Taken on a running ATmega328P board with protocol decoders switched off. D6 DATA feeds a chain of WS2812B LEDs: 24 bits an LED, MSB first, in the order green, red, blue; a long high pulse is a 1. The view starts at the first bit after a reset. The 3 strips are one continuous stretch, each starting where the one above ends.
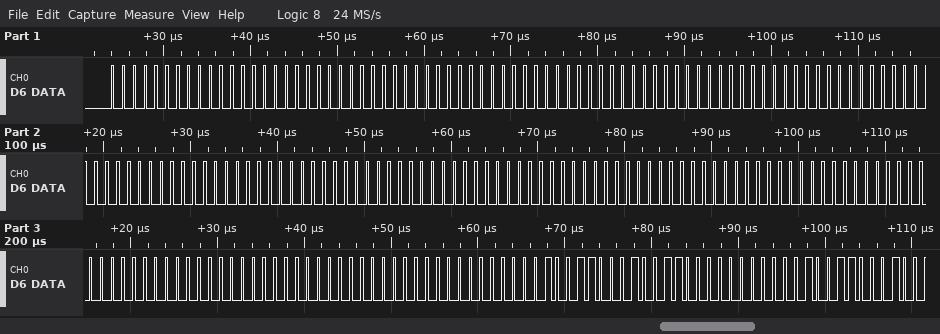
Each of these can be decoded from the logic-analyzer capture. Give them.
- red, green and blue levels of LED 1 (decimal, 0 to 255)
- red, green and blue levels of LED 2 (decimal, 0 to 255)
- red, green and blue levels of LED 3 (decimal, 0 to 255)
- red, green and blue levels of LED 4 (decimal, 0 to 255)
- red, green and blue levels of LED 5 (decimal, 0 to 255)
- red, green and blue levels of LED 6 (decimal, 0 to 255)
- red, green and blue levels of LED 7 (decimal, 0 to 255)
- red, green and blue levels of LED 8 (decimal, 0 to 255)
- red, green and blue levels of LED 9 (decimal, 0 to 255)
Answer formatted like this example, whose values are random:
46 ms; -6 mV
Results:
0, 0, 0; 0, 0, 0; 0, 0, 0; 0, 0, 0; 0, 0, 0; 0, 0, 0; 0, 0, 0; 0, 0, 0; 19, 19, 0
